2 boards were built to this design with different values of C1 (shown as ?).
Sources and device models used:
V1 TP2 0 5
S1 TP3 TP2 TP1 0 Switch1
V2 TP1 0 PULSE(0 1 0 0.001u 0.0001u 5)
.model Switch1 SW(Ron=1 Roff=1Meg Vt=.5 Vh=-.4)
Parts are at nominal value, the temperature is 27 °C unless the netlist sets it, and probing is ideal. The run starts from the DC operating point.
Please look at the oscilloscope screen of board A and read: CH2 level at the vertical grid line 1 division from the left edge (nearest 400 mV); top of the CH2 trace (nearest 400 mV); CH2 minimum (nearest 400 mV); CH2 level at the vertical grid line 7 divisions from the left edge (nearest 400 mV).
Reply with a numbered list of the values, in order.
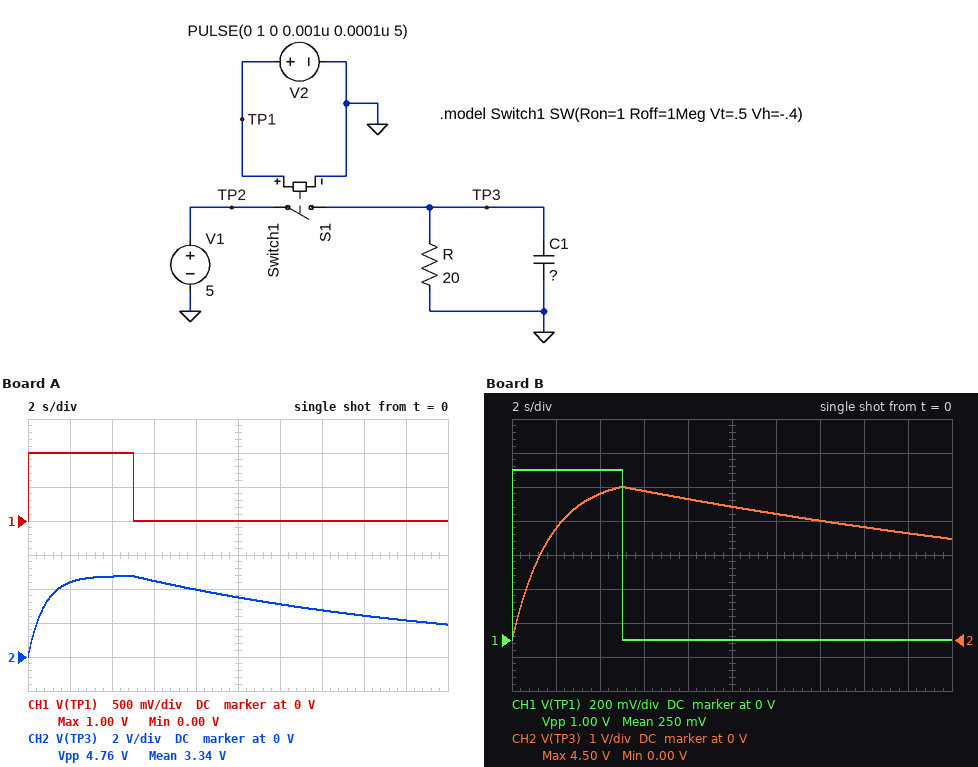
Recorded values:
1. 4.4 V
2. 4.8 V
3. 0 V
4. 2.8 V
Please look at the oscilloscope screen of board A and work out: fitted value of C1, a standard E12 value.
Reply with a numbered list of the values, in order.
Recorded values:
1. 820 mF
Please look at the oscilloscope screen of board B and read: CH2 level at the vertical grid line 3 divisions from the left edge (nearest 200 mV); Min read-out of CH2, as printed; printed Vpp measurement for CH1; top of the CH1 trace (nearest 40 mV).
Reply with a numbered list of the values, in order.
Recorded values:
1. 4.4 V
2. 0.00 V
3. 1.00 V
4. 1.00 V
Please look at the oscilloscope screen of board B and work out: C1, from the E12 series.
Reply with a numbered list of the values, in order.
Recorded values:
1. 1.8 F
